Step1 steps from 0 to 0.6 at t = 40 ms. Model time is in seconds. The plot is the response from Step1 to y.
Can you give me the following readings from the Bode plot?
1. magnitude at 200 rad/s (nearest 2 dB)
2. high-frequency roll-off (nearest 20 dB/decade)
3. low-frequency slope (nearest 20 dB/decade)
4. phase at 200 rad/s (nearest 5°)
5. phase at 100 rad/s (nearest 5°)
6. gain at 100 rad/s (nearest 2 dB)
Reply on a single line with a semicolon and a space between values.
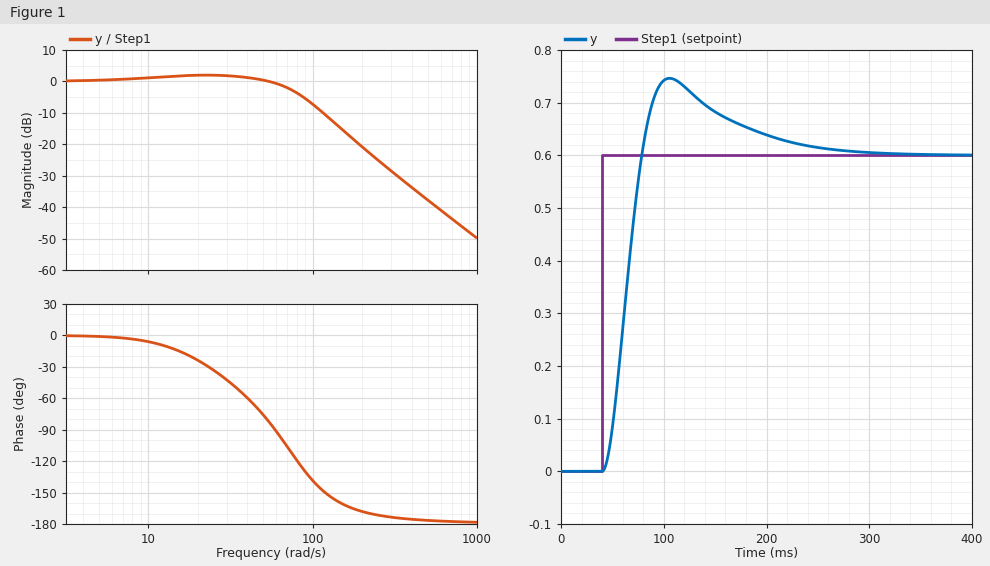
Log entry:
-20 dB; -40 dB/decade; 0 dB/decade; -170°; -140°; -8 dB
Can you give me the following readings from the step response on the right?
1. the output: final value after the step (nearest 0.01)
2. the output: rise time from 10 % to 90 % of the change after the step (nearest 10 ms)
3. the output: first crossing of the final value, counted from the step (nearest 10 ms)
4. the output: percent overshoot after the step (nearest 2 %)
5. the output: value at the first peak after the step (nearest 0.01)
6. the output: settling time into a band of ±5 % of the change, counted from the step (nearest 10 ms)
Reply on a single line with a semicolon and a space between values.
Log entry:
0.60; 30 ms; 40 ms; 24 %; 0.75; 170 ms
